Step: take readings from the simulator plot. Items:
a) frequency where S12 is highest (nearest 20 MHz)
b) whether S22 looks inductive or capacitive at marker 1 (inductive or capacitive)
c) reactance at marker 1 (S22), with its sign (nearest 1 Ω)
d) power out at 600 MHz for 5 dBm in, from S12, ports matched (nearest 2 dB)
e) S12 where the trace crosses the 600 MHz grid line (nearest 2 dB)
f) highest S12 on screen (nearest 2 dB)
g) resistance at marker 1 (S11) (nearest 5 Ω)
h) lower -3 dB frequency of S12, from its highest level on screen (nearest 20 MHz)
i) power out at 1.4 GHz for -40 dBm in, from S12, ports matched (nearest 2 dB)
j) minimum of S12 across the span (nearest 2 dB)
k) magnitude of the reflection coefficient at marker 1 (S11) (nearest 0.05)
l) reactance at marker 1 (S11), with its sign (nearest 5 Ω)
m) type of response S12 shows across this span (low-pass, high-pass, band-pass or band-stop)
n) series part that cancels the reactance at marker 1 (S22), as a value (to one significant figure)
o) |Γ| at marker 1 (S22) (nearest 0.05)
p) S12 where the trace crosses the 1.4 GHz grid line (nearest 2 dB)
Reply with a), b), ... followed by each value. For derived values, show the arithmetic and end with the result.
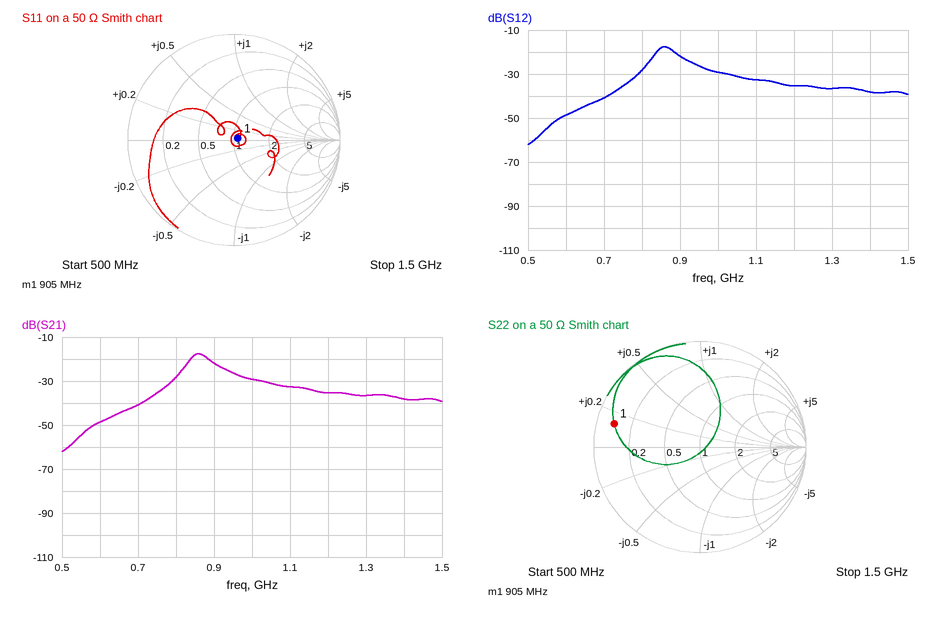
a) 860 MHz
b) inductive
c) +7 Ω
d) 5 dBm + (-48 dB) = -44 dBm
e) -48 dB
f) -18 dB
g) 55 Ω
h) 840 MHz
i) -40 dBm + (-38 dB) = -78 dBm
j) -62 dB
k) 0.05
l) 0 Ω
m) band-pass
n) C = 1/(2π × 905 MHz × 7 Ω) ≈ 25.1 pF, so 30 pF to one significant figure
o) 0.85
p) -38 dB
